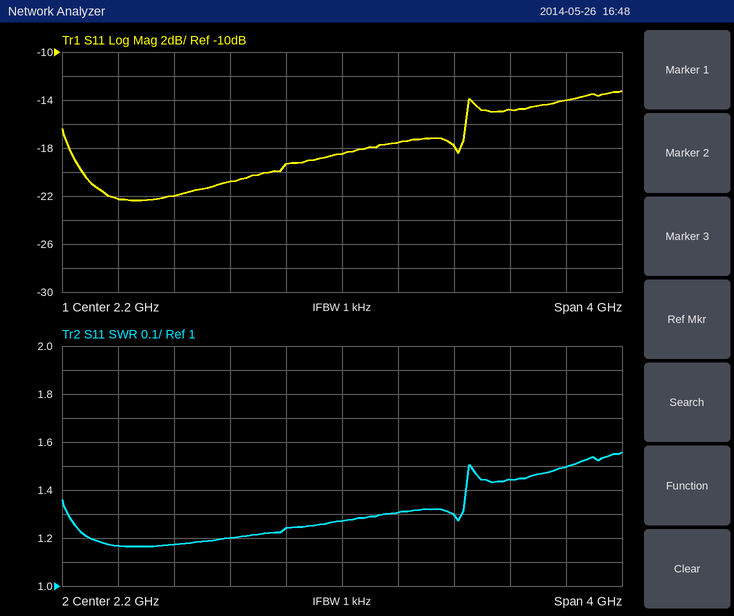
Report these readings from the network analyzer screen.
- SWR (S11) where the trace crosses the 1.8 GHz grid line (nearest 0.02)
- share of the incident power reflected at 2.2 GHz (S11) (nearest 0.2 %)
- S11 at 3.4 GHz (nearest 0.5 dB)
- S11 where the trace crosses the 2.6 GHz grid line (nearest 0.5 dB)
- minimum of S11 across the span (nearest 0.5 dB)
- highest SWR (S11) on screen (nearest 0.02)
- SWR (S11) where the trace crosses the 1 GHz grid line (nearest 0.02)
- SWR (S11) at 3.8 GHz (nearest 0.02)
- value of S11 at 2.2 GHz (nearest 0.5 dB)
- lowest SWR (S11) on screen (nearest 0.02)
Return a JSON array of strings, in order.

["1.24", "1.4 %", "-15.0 dB", "-17.5 dB", "-22.5 dB", "1.56", "1.18", "1.50", "-18.5 dB", "1.16"]
